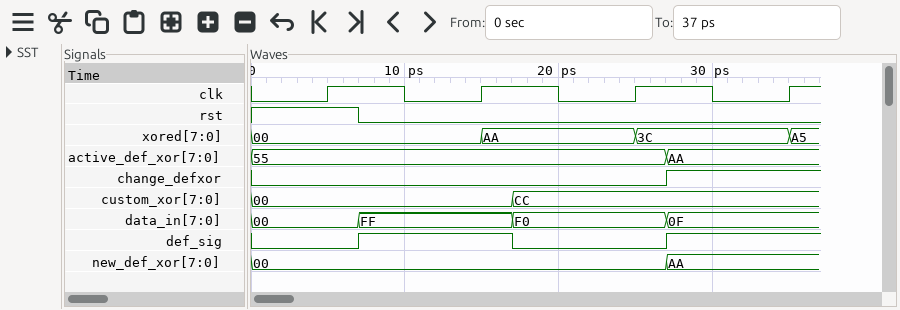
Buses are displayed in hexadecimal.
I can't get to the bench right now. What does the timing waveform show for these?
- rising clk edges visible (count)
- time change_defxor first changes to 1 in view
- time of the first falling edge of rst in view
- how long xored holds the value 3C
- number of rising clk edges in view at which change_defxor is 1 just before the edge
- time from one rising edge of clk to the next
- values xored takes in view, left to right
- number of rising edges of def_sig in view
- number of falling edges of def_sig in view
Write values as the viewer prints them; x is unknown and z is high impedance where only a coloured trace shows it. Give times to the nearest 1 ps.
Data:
4
27 ps
7 ps
10 ps
1
10 ps
00, AA, 3C, A5
2
1
